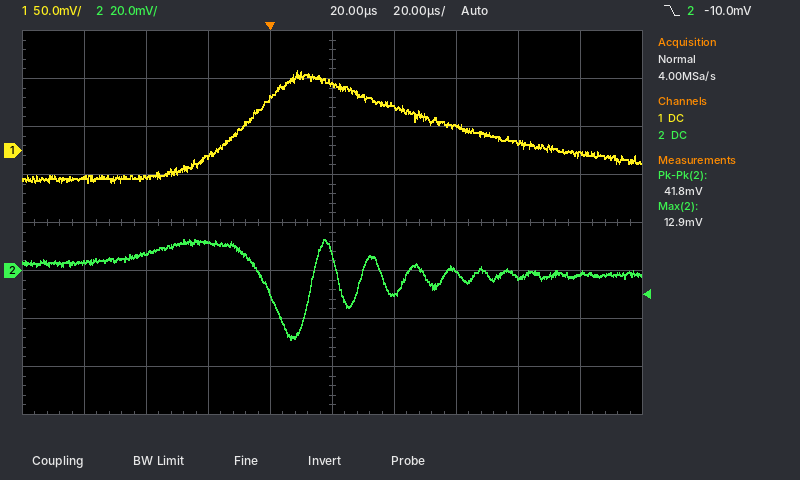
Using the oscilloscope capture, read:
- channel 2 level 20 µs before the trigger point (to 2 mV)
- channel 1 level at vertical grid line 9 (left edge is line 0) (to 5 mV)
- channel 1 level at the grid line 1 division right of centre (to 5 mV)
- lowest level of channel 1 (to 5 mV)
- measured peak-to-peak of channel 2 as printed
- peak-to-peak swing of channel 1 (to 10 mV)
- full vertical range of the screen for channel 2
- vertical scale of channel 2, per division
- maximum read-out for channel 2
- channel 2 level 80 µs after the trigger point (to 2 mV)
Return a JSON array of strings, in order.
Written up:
["12 mV", "-5 mV", "45 mV", "-35 mV", "41.8 mV", "120 mV", "160 mV", "20 mV", "12.9 mV", "-2 mV"]
